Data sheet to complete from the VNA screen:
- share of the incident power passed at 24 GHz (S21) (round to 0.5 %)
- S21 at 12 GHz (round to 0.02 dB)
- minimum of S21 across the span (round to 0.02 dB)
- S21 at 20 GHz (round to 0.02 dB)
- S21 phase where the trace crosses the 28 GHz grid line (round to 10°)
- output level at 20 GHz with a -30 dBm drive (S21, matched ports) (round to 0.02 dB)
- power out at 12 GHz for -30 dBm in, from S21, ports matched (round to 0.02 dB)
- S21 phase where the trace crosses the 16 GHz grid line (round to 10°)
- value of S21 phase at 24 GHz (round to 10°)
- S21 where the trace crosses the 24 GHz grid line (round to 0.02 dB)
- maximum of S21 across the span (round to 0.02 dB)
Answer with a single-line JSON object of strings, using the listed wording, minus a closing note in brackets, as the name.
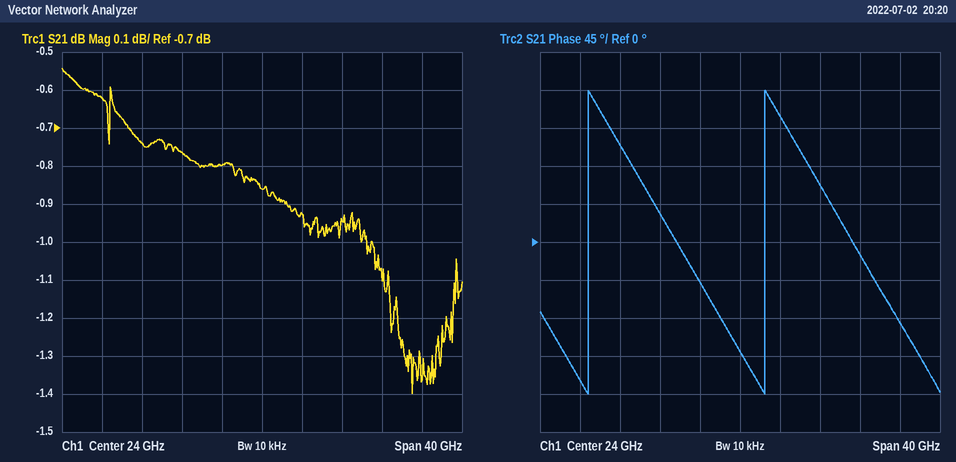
{"share of the incident power passed at 24 GHz (S21)": "82.0 %", "S21 at 12 GHz": "-0.74 dB", "minimum of S21 across the span": "-1.40 dB", "S21 at 20 GHz": "-0.80 dB", "S21 phase where the trace crosses the 28 GHz grid line": "150°", "output level at 20 GHz with a -30 dBm drive (S21, matched ports)": "-30.80 dBm", "power out at 12 GHz for -30 dBm in, from S21, ports matched": "-30.74 dBm", "S21 phase where the trace crosses the 16 GHz grid line": "30°", "value of S21 phase at 24 GHz": "-130°", "S21 where the trace crosses the 24 GHz grid line": "-0.86 dB", "maximum of S21 across the span": "-0.54 dB"}
